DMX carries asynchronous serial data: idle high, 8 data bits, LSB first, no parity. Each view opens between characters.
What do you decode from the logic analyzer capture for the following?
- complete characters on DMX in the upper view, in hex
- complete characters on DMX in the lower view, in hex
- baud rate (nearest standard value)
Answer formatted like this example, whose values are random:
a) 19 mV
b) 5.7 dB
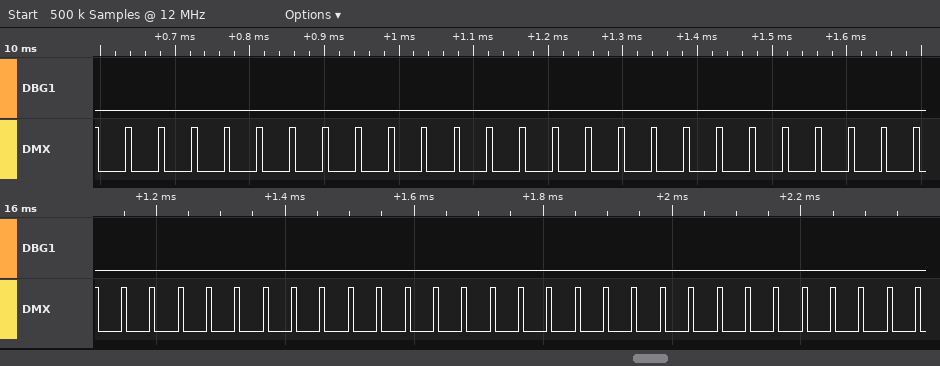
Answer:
a) 08, 08, 08, 08, 08, 08, 08, 08, 08, 08, 08, 08
b) 08, 08, 08, 08, 08, 08, 08, 08, 08, 08, 08, 08, 08, 08
c) 115200 baud
